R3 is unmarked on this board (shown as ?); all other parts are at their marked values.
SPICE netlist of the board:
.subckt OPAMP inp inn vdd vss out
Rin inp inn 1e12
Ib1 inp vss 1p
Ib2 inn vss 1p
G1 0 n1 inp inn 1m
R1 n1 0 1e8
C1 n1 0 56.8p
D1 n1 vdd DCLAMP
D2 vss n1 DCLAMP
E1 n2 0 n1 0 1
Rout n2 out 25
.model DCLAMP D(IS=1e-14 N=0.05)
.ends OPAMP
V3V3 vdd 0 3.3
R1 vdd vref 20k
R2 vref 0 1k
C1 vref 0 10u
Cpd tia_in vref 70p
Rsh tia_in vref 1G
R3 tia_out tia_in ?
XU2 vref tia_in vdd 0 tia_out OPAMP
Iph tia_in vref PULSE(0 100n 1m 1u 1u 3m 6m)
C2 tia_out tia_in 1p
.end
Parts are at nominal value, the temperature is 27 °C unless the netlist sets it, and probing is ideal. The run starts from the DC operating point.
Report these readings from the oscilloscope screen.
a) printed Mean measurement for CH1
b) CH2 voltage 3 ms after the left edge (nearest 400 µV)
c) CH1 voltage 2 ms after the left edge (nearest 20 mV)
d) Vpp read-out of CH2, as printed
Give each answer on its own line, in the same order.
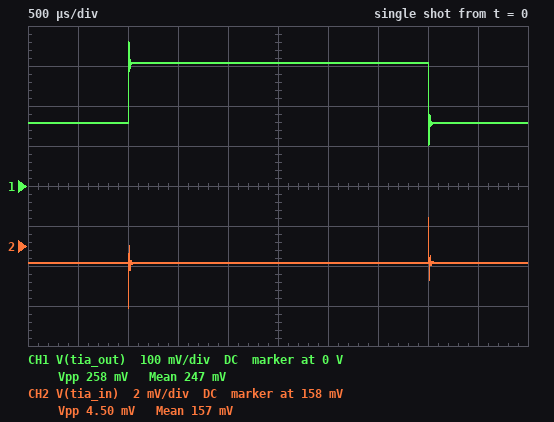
247 mV
157.2 mV
300 mV
4.50 mV
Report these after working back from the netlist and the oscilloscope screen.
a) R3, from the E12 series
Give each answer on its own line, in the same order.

1.5 MΩ
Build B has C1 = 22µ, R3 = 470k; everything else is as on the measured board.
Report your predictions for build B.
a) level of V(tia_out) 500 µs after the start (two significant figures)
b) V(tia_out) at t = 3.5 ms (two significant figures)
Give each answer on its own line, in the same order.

160 mV
200 mV
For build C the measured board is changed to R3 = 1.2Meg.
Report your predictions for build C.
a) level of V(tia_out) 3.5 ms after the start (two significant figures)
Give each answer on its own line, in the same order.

280 mV
